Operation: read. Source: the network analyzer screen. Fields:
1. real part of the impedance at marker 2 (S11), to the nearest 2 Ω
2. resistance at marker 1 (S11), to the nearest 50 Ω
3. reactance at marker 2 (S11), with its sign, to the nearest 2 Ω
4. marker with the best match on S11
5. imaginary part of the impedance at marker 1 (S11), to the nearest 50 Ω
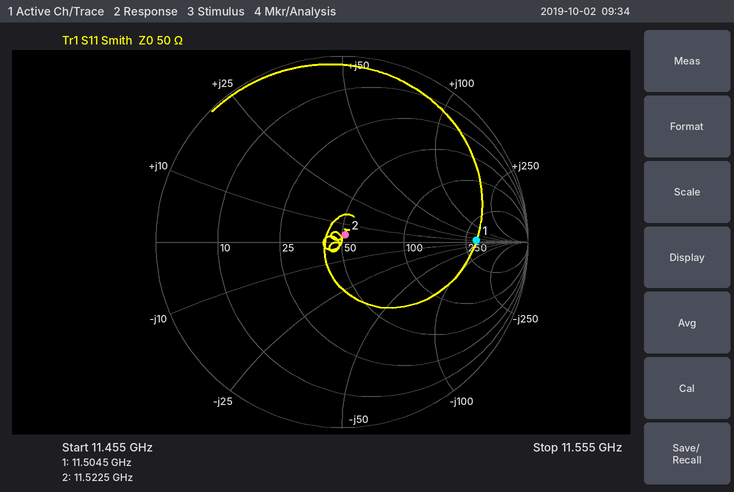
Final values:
52 Ω
300 Ω
+4 Ω
marker 2
0 Ω
